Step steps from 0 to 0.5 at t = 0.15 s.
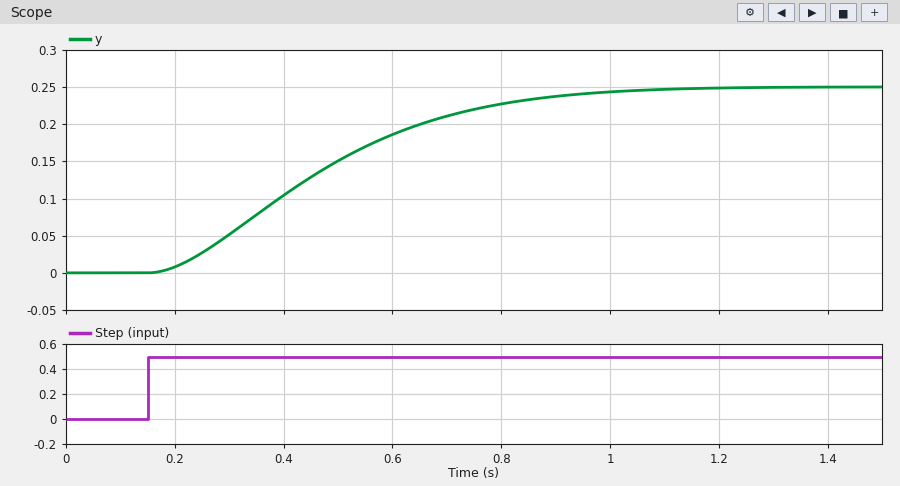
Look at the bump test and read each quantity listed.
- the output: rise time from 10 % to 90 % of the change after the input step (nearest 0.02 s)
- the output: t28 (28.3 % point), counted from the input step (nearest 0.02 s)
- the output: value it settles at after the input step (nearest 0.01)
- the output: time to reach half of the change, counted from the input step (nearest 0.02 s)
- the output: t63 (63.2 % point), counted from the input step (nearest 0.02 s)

0.54 s
0.18 s
0.25
0.30 s
0.36 s
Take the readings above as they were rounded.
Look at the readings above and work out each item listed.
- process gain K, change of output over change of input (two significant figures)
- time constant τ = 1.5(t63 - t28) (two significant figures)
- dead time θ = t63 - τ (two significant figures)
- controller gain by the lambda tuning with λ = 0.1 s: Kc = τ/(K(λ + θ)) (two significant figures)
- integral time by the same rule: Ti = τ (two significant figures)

0.50
0.27 s
0.090 s
2.8
0.27 s
